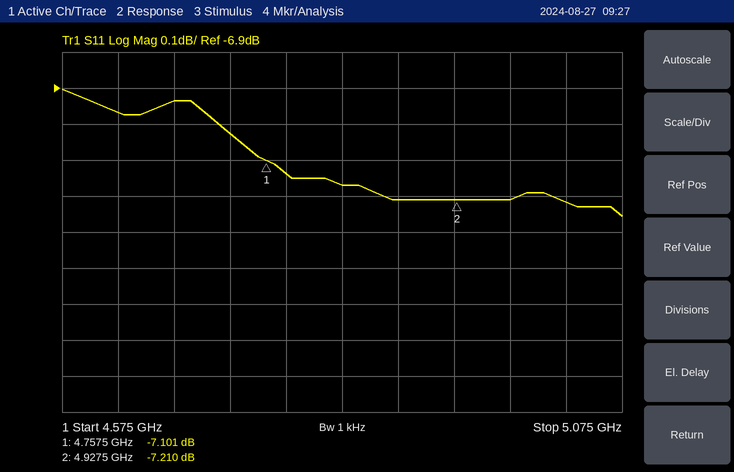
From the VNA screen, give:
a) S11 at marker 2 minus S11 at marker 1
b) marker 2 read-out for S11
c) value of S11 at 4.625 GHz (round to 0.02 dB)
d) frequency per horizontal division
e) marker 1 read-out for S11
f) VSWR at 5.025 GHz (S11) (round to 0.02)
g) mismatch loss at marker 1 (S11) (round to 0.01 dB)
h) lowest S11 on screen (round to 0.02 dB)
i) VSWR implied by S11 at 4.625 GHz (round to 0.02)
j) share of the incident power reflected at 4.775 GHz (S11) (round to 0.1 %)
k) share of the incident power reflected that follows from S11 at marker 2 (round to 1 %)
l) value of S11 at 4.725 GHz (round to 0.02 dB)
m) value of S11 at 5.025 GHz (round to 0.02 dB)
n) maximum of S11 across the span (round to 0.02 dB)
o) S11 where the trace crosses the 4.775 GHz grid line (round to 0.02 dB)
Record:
-0.109 dB
-7.210 dB
-6.96 dB
50 MHz
-7.101 dB
2.54
0.94 dB
-7.26 dB
2.62
19.3 %
19 %
-7.02 dB
-7.22 dB
-6.90 dB
-7.14 dB
